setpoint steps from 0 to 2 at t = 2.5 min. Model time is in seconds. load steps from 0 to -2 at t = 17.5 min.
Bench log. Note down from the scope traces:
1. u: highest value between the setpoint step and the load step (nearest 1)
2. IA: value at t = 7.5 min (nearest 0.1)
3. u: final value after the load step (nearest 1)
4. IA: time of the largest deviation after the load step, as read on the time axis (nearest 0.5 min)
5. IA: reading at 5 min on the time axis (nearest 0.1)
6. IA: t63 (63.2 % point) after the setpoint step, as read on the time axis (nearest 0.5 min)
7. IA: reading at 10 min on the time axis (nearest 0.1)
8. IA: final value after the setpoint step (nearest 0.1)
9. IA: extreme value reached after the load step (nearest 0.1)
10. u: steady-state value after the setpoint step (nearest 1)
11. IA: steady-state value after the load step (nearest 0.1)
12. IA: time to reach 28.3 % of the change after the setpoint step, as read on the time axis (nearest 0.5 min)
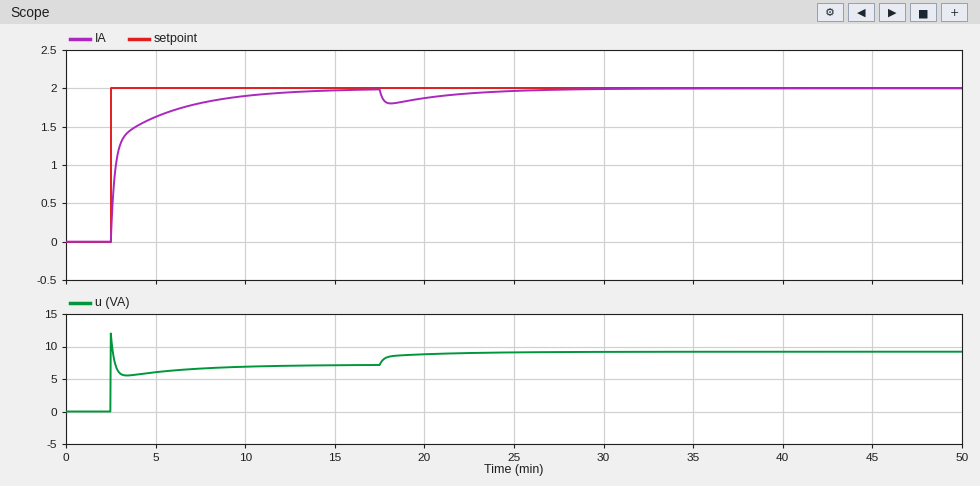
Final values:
12
1.8
9
18.0 min
1.6
3.0 min
1.9
2.0
1.8
7
2.0
2.5 min
